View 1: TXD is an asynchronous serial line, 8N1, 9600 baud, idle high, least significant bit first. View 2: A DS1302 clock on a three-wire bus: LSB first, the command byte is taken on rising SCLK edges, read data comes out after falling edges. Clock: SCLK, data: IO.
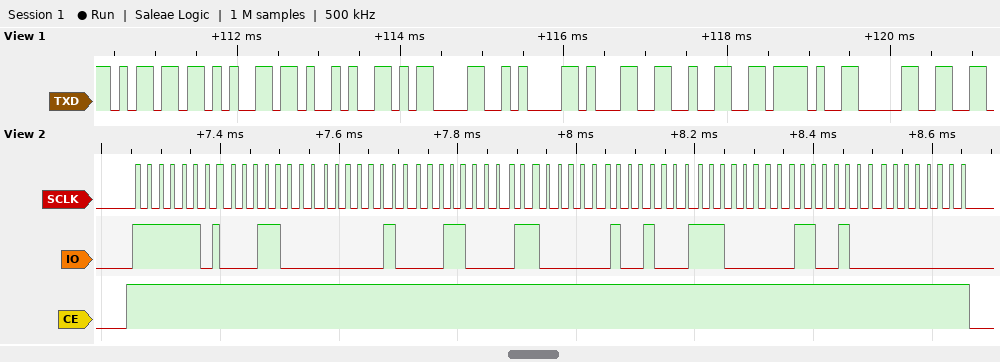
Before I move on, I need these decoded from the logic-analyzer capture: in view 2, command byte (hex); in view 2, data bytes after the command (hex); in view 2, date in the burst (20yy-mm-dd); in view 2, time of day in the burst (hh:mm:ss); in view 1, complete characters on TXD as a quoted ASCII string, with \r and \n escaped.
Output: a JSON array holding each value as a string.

["0xBF", "18 40 18 06 12 07 26 00", "2026-12-06", "18:40:18", "\"me)\\r\\n12/0\""]
